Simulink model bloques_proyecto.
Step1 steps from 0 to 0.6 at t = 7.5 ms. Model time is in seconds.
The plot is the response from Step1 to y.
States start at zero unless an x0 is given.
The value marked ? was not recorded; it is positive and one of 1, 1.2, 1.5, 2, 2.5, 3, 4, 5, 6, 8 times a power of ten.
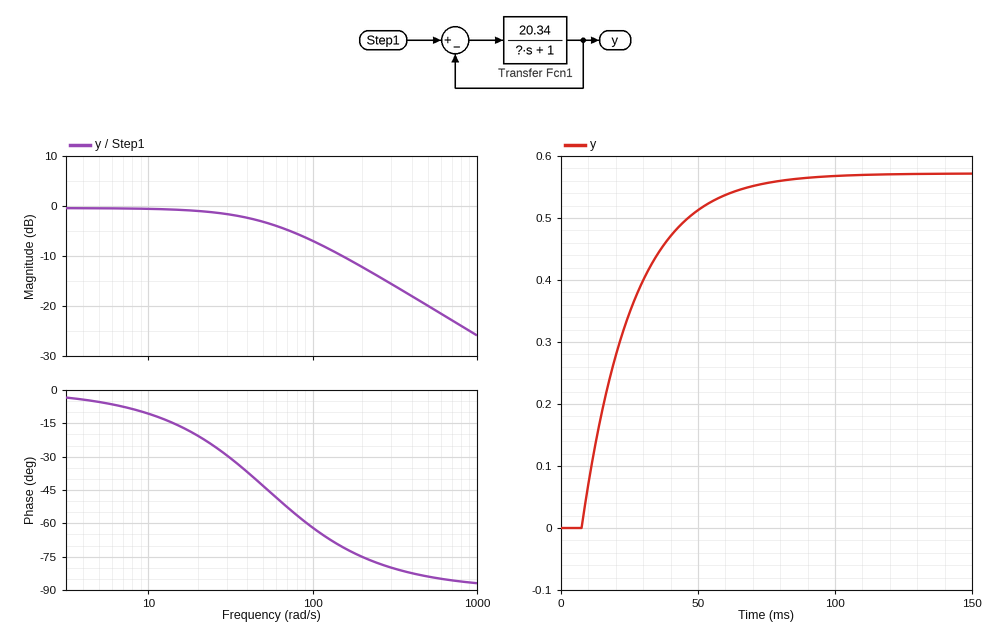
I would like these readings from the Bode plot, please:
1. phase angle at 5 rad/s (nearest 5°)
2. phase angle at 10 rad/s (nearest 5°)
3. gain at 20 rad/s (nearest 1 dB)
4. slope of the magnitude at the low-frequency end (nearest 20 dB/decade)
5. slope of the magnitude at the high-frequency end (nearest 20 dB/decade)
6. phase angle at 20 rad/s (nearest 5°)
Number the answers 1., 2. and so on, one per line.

1. -5°
2. -10°
3. -1 dB
4. 0 dB/decade
5. -20 dB/decade
6. -20°
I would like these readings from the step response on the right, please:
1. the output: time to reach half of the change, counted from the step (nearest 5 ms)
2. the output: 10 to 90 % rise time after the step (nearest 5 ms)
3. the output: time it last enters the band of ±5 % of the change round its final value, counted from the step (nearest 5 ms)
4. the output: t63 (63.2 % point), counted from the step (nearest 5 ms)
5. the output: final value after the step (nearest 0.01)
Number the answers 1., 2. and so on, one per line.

1. 15 ms
2. 40 ms
3. 55 ms
4. 20 ms
5. 0.57
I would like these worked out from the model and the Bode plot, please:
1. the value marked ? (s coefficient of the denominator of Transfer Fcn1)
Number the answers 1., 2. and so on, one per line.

1. 0.4
